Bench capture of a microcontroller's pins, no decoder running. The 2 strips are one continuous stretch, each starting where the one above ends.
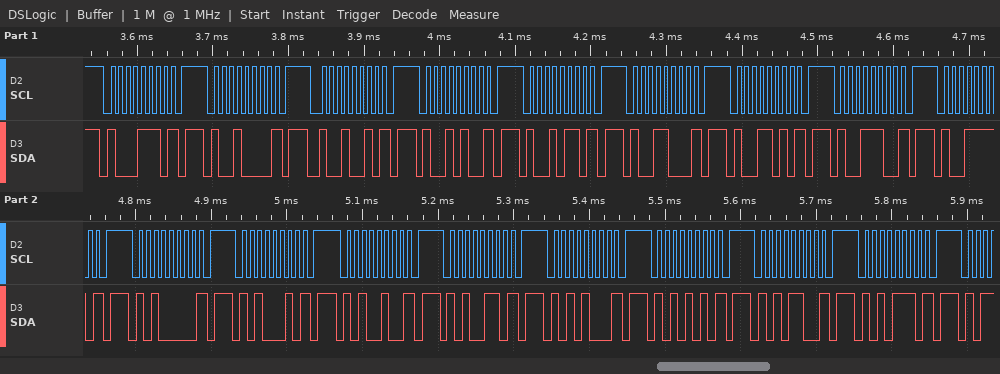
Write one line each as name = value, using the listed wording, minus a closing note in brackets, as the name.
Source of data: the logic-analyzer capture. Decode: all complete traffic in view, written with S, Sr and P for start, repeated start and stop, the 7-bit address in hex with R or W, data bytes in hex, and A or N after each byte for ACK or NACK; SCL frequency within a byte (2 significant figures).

all complete traffic in view, written with S, Sr and P for start, repeated start and stop, the 7-bit address in hex with R or W, data bytes in hex, and A or N after each byte for ACK or NACK = S 47W N P S 48W N P S 49W N P S 4AW N P S 4BW N P S 4CW N P S 4DW N P S 4EW N P S 4FW N P S 50W N P S 51W N P S 52W N P S 53W N P S 54W N P S 55W N P S 56W N P S 57W N P
SCL frequency within a byte = 100 kHz
